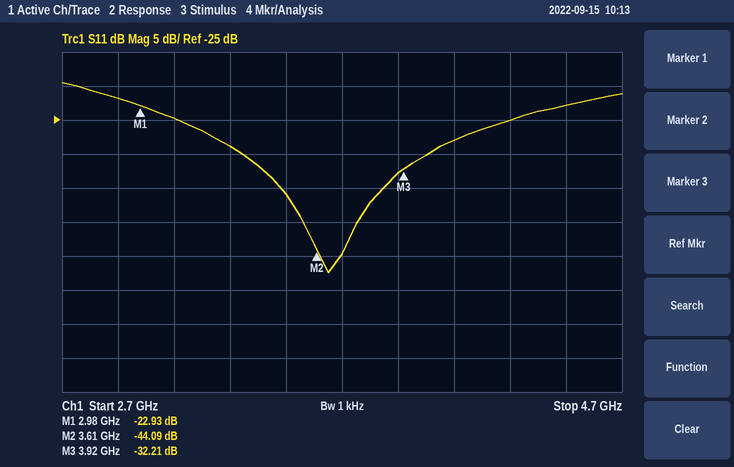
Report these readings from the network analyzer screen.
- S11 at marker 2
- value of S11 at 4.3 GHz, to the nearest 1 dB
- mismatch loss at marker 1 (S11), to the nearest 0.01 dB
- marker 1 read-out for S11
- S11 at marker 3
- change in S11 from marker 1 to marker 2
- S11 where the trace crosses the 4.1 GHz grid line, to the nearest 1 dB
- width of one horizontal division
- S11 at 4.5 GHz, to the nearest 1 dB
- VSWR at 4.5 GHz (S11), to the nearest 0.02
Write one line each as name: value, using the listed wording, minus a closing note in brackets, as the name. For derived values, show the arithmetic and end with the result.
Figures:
S11 at marker 2: -44.09 dB
value of S11 at 4.3 GHz, to the nearest 1 dB: -25 dB
mismatch loss at marker 1 (S11), to the nearest 0.01 dB: −10 log10(1 − 10^(-22.93/10)) ≈ 0.02 dB
marker 1 read-out for S11: -22.93 dB
S11 at marker 3: -32.21 dB
change in S11 from marker 1 to marker 2: -44.09 − (-22.93) = -21.16 dB
S11 where the trace crosses the 4.1 GHz grid line, to the nearest 1 dB: -28 dB
width of one horizontal division: 200 MHz
S11 at 4.5 GHz, to the nearest 1 dB: -23 dB
VSWR at 4.5 GHz (S11), to the nearest 0.02: |Γ| = 10^(-23/20) = 0.0708; VSWR = (1 + 0.0708)/(1 − 0.0708) ≈ 1.15, so 1.16 to the nearest 0.02
